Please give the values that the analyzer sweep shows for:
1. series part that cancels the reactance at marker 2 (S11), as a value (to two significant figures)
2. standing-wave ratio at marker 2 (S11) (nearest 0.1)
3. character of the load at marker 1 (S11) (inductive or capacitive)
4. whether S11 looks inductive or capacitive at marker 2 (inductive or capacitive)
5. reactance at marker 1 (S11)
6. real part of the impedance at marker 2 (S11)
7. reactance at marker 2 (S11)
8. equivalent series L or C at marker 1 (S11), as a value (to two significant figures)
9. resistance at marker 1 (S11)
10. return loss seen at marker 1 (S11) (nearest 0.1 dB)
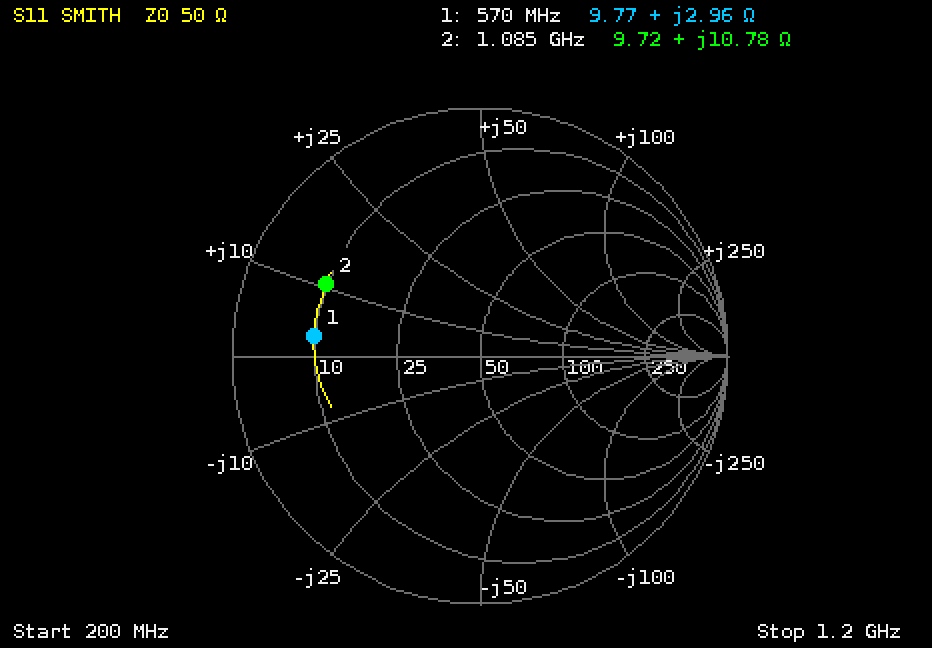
14 pF
5.4
inductive
inductive
+2.96 Ω
9.72 Ω
+10.78 Ω
830 pH
9.77 Ω
3.4 dB
